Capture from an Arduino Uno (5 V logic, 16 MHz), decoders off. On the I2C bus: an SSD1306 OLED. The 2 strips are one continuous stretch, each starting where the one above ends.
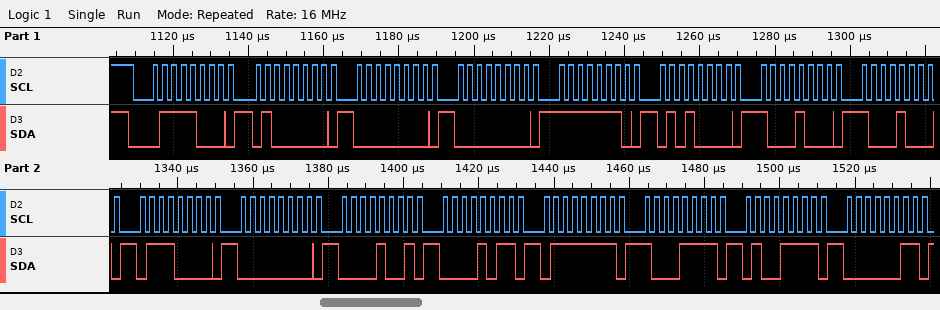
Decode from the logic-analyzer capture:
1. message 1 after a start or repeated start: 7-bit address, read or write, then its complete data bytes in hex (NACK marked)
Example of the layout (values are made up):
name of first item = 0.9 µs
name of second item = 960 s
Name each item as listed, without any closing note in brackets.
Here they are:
message 1 after a start or repeated start: 7-bit address, read or write, then its complete data bytes in hex = 0x3C write: 40 00 00 FE 50 88 88 70 00 09 0B 7F 8F 4F 03
